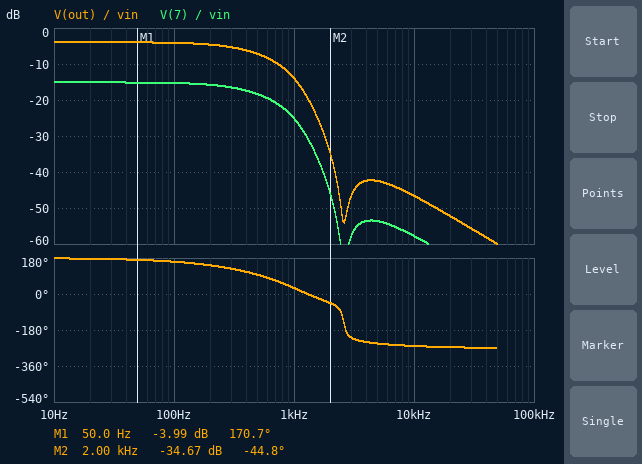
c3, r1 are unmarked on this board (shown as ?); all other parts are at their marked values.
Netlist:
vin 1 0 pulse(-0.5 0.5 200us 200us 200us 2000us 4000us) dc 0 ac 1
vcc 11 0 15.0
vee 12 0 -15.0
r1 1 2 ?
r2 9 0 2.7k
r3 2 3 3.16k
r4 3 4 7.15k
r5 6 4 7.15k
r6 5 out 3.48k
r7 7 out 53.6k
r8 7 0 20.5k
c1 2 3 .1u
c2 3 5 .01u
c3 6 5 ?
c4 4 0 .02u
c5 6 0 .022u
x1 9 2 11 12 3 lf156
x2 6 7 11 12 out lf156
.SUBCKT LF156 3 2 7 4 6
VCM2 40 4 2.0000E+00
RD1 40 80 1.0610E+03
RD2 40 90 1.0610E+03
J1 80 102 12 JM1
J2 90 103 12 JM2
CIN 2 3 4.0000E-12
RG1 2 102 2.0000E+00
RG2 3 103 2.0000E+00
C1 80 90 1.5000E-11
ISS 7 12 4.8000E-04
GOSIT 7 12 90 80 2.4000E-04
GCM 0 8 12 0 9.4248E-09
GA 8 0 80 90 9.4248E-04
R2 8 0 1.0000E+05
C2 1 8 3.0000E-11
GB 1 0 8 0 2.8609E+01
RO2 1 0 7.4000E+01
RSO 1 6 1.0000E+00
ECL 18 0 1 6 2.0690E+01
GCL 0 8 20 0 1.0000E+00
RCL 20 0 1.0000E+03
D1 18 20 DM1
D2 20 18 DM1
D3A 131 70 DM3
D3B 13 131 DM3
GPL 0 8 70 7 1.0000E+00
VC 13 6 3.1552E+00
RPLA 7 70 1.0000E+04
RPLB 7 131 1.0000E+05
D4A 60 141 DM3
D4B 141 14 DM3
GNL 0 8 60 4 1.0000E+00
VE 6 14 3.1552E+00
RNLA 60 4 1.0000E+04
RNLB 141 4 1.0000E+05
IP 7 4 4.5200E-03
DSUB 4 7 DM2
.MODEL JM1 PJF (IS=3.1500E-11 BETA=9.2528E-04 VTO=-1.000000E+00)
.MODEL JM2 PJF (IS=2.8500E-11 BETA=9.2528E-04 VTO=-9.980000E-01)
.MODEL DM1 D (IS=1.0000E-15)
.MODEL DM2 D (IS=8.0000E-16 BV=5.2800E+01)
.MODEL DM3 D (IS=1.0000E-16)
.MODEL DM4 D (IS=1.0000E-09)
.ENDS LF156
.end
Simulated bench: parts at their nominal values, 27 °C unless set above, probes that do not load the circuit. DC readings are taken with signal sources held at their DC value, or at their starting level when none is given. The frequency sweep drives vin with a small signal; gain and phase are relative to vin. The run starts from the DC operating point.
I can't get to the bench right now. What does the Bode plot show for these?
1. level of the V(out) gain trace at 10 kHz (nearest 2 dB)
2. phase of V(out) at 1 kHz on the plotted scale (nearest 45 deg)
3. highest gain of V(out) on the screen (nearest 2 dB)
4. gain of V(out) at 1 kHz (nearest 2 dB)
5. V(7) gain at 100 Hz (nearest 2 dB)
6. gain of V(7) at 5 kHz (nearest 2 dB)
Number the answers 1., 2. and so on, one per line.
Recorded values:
1. -46 dB
2. 45 deg
3. -4 dB
4. -14 dB
5. -16 dB
6. -54 dB
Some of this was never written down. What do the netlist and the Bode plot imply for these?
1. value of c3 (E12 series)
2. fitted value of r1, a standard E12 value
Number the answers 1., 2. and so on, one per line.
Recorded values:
1. 6.8 nF
2. 18 kΩ
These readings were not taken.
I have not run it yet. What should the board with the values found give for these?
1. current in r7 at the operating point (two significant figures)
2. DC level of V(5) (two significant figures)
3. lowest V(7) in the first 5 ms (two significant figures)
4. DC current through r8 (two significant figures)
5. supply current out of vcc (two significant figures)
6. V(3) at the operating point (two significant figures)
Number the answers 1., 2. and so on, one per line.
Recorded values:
1. 210 nA
2. 16 mV
3. -83 mV
4. 210 nA
5. 10 mA
6. 2.4 mV
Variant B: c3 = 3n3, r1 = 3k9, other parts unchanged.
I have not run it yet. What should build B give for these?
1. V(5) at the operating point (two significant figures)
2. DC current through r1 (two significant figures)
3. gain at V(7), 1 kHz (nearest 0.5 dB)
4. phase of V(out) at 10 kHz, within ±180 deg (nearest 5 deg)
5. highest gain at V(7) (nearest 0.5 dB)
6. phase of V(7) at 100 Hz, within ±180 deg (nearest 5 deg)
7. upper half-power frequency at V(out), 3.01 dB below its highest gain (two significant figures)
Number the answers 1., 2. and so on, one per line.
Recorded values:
1. 20 mV
2. 510 nA
3. -15.5 dB
4. 110 deg
5. -2.0 dB
6. 155 deg
7. 350 Hz
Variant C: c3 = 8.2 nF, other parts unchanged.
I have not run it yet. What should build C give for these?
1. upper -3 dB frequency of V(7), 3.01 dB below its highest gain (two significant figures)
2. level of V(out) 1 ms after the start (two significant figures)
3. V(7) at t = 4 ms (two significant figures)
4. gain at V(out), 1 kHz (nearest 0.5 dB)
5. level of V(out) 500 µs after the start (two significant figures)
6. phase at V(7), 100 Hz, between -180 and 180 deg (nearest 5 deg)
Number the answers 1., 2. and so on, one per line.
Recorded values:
1. 590 Hz
2. -210 mV
3. 89 mV
4. -11.5 dB
5. 240 mV
6. 165 deg
